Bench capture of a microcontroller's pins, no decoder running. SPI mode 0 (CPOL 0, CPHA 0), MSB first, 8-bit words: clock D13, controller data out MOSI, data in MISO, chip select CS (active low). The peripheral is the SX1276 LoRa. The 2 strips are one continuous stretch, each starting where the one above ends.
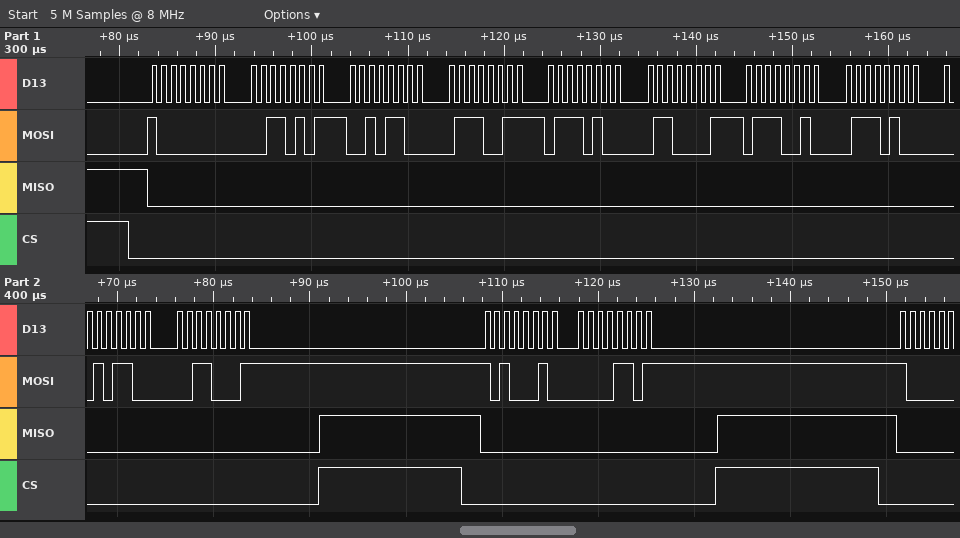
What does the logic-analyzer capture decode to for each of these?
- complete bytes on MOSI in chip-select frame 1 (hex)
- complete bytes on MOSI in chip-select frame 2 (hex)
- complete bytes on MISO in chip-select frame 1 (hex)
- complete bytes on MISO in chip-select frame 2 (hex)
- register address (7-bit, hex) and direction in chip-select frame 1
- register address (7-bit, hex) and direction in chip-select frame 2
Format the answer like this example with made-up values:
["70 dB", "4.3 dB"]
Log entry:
["80 35 2C 73 74 61 72 74 2C 31", "A2 0D", "00 00 00 00 00 00 00 00 00 00", "00 00", "0x00 write", "0x22 write"]
